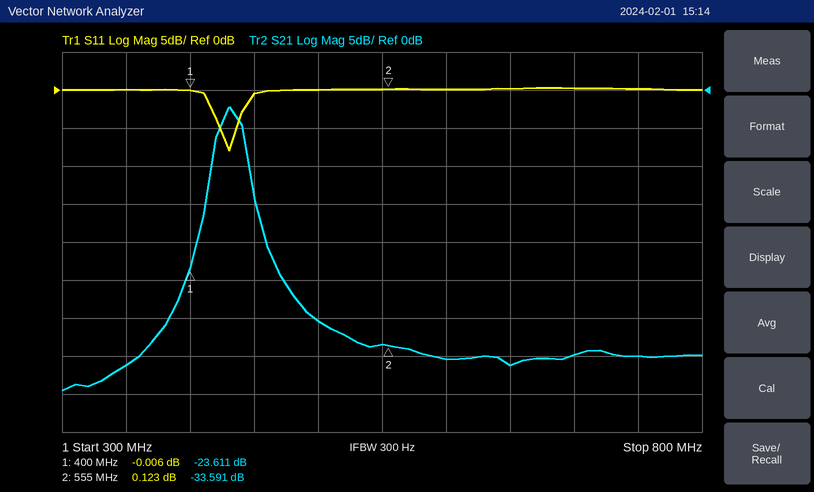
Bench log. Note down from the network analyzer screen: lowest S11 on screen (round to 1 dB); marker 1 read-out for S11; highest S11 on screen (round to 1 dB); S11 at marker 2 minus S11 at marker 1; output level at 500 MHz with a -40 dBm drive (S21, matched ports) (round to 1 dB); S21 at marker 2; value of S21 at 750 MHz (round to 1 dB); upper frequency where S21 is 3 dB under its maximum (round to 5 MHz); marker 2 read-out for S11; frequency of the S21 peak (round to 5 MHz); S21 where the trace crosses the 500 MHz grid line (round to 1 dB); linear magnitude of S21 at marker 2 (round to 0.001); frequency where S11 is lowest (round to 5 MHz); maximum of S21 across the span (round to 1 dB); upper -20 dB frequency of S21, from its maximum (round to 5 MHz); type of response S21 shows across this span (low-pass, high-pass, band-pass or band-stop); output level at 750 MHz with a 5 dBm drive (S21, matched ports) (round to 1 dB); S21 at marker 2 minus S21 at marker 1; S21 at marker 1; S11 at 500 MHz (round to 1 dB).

-8 dB
-0.006 dB
0 dB
0.129 dB
-70 dBm
-33.591 dB
-35 dB
440 MHz
0.123 dB
430 MHz
-30 dB
0.021
430 MHz
-2 dB
465 MHz
band-pass
-30 dBm
-9.980 dB
-23.611 dB
0 dB
